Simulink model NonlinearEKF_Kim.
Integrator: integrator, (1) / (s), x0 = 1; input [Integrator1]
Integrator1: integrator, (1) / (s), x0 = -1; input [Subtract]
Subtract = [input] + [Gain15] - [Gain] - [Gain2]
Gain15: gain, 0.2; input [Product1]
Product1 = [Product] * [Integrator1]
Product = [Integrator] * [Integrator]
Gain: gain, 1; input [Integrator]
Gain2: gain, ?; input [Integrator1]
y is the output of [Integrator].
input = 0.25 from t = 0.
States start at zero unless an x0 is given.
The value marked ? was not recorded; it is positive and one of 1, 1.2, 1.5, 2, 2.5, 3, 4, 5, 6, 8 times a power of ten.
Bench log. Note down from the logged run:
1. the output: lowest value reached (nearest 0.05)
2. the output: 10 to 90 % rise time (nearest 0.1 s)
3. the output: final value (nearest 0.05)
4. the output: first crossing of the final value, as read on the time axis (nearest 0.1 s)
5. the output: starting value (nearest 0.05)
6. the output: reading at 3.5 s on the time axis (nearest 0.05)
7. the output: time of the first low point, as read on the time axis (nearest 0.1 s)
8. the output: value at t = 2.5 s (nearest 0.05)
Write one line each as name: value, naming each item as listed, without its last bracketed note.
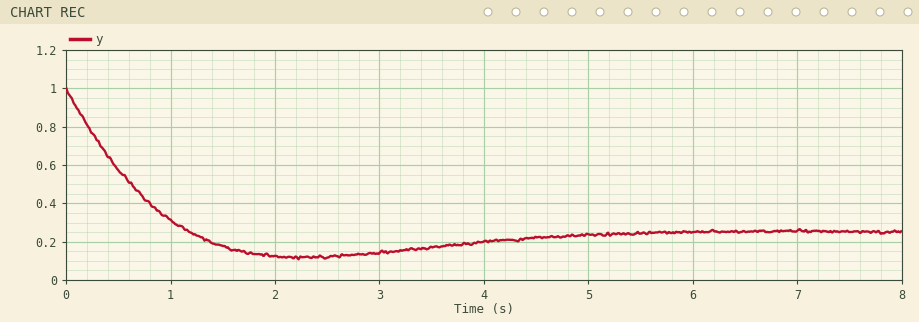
the output: lowest value reached: 0.10
the output: 10 to 90 % rise time: 0.9 s
the output: final value: 0.25
the output: first crossing of the final value, as read on the time axis: 1.2 s
the output: starting value: 1.00
the output: reading at 3.5 s on the time axis: 0.15
the output: time of the first low point, as read on the time axis: 2.3 s
the output: value at t = 2.5 s: 0.10
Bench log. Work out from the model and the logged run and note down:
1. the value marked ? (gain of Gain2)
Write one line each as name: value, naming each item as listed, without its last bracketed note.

the value marked ?: 1.5
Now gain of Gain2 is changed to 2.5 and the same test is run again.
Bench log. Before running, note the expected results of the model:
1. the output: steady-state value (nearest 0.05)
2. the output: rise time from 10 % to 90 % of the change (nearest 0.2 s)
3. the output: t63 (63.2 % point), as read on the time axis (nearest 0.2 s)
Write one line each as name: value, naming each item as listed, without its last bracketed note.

the output: steady-state value: 0.25
the output: rise time from 10 % to 90 % of the change: 2.6 s
the output: t63 (63.2 % point), as read on the time axis: 0.8 s
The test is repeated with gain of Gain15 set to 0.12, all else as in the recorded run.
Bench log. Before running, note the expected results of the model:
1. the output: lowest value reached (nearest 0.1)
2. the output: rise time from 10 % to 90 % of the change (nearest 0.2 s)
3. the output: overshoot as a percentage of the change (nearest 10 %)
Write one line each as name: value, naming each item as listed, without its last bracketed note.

the output: lowest value reached: 0.1
the output: rise time from 10 % to 90 % of the change: 1.0 s
the output: overshoot as a percentage of the change: 20 %
